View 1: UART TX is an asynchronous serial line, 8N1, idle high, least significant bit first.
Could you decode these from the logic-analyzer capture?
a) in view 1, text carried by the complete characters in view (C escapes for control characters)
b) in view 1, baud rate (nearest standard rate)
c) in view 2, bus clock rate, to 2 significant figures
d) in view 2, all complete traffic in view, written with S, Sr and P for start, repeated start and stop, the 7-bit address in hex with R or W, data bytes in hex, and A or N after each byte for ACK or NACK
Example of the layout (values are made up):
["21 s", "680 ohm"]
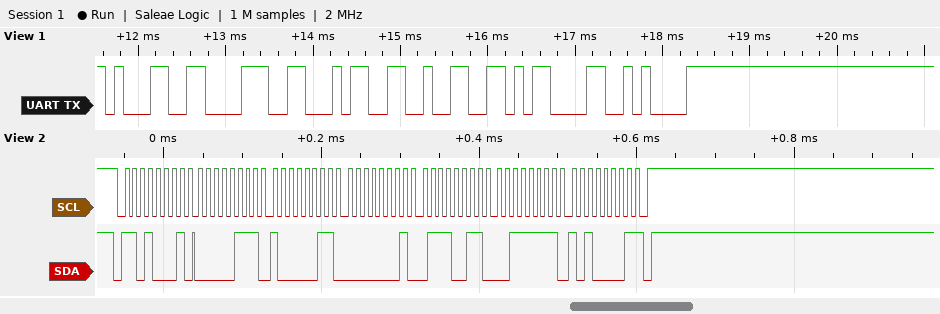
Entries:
["\"1842\\r\\n\"", "9600 baud", "100 kHz", "S 68R A 07 A 83 A 01 A 73 A 3F A A1 N P"]
